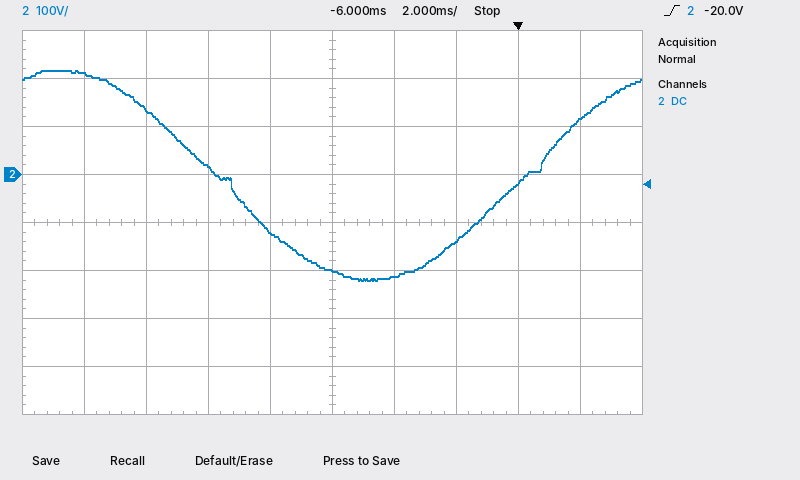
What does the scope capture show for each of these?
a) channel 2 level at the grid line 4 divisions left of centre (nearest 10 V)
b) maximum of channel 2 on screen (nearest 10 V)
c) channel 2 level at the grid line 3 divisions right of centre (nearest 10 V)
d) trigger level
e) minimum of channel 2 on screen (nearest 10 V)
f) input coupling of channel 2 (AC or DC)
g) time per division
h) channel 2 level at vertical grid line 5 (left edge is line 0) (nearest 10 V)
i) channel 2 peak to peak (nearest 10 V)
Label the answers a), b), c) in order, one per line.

a) 210 V
b) 220 V
c) -20 V
d) -20.0 V
e) -220 V
f) DC
g) 2 ms
h) -200 V
i) 440 V
